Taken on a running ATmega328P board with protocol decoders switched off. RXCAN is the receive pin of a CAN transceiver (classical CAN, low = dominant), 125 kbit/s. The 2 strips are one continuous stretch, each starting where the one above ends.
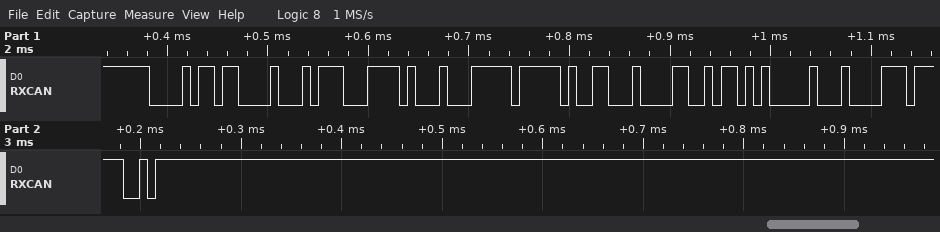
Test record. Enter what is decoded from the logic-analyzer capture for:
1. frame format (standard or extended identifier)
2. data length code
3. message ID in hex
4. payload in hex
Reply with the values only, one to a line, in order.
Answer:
standard
8
0x0B6
B8 F4 47 FF 31 0C B5 00
